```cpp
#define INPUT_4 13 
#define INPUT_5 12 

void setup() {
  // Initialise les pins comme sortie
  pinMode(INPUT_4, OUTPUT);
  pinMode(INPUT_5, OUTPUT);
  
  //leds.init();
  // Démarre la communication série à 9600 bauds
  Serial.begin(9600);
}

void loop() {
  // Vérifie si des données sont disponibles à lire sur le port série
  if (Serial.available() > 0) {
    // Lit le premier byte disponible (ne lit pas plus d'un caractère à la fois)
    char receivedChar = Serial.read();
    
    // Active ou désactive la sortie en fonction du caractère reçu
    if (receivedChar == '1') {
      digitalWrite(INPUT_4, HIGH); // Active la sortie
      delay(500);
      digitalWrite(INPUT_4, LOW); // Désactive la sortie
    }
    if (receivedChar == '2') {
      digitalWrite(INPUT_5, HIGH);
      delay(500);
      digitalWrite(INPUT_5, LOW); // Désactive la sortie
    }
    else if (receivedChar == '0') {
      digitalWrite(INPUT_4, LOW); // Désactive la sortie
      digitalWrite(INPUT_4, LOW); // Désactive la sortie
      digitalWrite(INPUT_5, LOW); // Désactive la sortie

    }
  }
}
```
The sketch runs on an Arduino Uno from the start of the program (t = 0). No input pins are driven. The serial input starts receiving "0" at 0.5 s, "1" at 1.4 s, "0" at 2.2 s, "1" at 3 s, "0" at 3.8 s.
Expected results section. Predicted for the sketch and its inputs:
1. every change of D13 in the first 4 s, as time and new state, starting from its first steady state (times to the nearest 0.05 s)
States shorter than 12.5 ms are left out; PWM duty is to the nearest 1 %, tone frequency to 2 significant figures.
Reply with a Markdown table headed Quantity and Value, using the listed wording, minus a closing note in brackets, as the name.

| Quantity | Value |
|---|---|
| every change of D13 in the first 4 s, as time and new state, starting from its first steady state | 0 s low; 1.4 s high; 1.9 s low; 3 s high; 3.5 s low |
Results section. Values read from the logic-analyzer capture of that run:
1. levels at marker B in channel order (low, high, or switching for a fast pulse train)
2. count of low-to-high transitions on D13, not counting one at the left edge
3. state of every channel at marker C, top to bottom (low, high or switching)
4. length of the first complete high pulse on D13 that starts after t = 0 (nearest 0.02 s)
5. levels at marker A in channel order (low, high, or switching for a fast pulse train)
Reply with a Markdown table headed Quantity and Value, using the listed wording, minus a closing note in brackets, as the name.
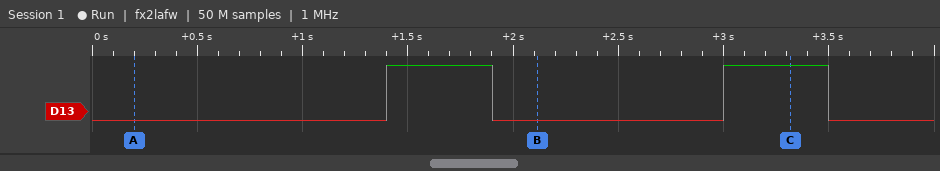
| Quantity | Value |
|---|---|
| levels at marker B in channel order | D13 low |
| count of low-to-high transitions on D13, not counting one at the left edge | 2 |
| state of every channel at marker C, top to bottom | D13 high |
| length of the first complete high pulse on D13 that starts after t = 0 | 0.50 s |
| levels at marker A in channel order | D13 low |
